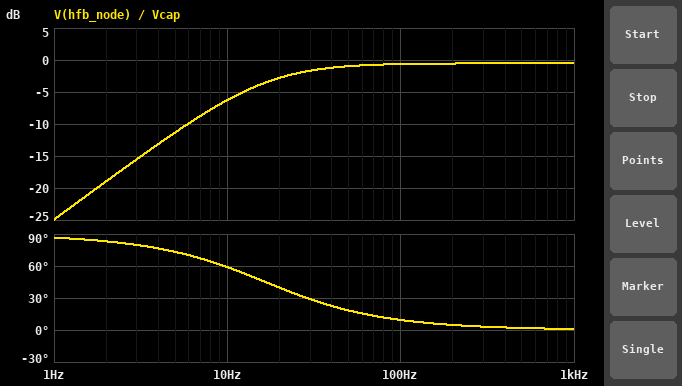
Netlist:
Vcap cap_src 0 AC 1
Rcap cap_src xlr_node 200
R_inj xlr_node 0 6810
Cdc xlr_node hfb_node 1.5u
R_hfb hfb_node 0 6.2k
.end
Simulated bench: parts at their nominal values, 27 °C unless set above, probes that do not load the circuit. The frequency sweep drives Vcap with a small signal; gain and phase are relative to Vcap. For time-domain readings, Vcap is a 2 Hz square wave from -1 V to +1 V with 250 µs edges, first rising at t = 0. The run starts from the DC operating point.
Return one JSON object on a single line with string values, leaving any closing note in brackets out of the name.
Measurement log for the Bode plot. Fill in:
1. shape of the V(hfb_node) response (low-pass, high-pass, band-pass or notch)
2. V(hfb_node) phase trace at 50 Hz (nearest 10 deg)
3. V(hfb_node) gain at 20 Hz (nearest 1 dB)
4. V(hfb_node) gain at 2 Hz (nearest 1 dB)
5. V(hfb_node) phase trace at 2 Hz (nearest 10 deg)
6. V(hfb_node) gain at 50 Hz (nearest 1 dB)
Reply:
{"shape of the V(hfb_node) response": "high-pass", "V(hfb_node) phase trace at 50 Hz": "20 deg", "V(hfb_node) gain at 20 Hz": "-3 dB", "V(hfb_node) gain at 2 Hz": "-19 dB", "V(hfb_node) phase trace at 2 Hz": "80 deg", "V(hfb_node) gain at 50 Hz": "-1 dB"}
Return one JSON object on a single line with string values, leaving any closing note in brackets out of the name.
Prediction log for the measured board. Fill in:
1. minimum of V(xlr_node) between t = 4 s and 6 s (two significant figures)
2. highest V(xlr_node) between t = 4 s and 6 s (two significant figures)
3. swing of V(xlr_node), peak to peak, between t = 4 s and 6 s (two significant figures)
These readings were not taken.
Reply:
{"minimum of V(xlr_node) between t = 4 s and 6 s": "-970 mV", "highest V(xlr_node) between t = 4 s and 6 s": "970 mV", "swing of V(xlr_node), peak to peak, between t = 4 s and 6 s": "1.9 V"}
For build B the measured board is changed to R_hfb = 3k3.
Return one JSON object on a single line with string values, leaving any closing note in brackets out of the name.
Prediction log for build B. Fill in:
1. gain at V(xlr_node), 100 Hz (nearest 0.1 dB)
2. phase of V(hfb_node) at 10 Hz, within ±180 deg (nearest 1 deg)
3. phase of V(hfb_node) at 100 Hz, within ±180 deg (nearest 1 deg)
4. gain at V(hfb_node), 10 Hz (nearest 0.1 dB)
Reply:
{"gain at V(xlr_node), 100 Hz": "-0.7 dB", "phase of V(hfb_node) at 10 Hz, within ±180 deg": "72 deg", "phase of V(hfb_node) at 100 Hz, within ±180 deg": "17 deg", "gain at V(hfb_node), 10 Hz": "-10.8 dB"}
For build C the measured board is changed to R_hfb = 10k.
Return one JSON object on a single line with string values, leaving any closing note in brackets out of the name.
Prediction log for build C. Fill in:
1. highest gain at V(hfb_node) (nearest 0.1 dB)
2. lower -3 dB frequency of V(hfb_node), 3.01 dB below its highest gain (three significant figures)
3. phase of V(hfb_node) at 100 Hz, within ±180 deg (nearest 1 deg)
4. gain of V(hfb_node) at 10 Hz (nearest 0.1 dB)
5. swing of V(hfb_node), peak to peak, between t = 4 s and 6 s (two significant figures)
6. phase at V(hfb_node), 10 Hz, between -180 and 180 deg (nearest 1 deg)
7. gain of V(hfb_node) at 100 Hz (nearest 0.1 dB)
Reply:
{"highest gain at V(hfb_node)": "-0.4 dB", "lower -3 dB frequency of V(hfb_node), 3.01 dB below its highest gain": "10.4 Hz", "phase of V(hfb_node) at 100 Hz, within ±180 deg": "6 deg", "gain of V(hfb_node) at 10 Hz": "-3.6 dB", "swing of V(hfb_node), peak to peak, between t = 4 s and 6 s": "3.8 V", "phase at V(hfb_node), 10 Hz, between -180 and 180 deg": "46 deg", "gain of V(hfb_node) at 100 Hz": "-0.5 dB"}
